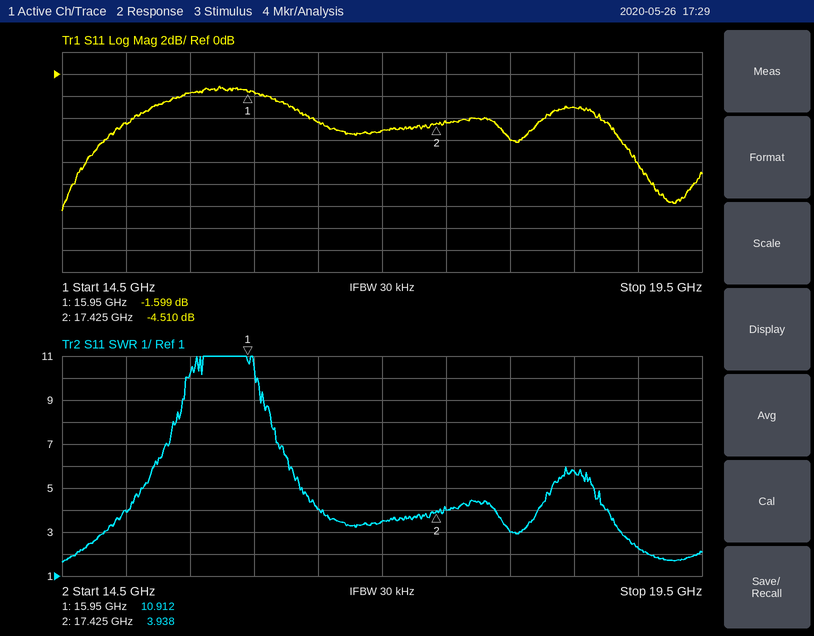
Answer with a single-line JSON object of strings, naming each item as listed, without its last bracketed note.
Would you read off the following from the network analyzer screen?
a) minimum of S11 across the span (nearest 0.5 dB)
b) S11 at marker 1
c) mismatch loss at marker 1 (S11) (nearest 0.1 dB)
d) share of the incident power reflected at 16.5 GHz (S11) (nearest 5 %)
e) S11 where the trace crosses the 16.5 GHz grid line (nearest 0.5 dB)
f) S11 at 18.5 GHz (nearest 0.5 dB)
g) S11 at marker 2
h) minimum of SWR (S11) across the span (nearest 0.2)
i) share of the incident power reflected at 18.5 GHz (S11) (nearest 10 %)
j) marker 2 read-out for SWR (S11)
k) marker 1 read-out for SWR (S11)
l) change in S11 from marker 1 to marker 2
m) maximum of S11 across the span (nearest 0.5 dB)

{"minimum of S11 across the span": "-12.5 dB", "S11 at marker 1": "-1.599 dB", "mismatch loss at marker 1 (S11)": "5.1 dB", "share of the incident power reflected at 16.5 GHz (S11)": "35 %", "S11 where the trace crosses the 16.5 GHz grid line": "-4.5 dB", "S11 at 18.5 GHz": "-3.0 dB", "S11 at marker 2": "-4.510 dB", "minimum of SWR (S11) across the span": "1.6", "share of the incident power reflected at 18.5 GHz (S11)": "50 %", "marker 2 read-out for SWR": "3.938", "marker 1 read-out for SWR": "10.912", "change in S11 from marker 1 to marker 2": "-2.911 dB", "maximum of S11 across the span": "-1.0 dB"}
